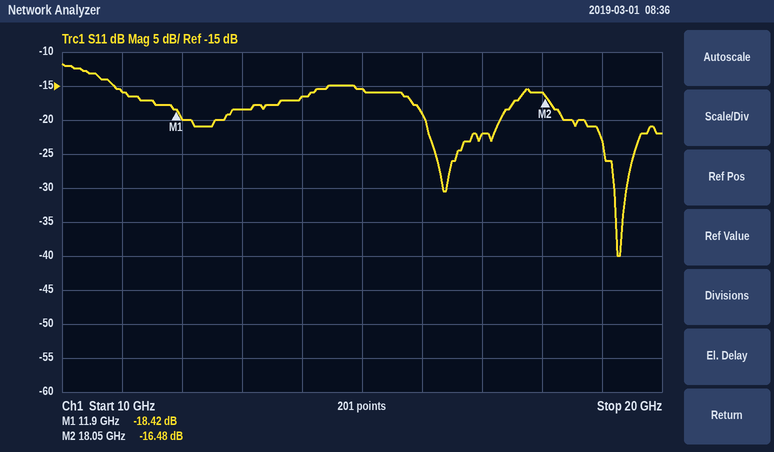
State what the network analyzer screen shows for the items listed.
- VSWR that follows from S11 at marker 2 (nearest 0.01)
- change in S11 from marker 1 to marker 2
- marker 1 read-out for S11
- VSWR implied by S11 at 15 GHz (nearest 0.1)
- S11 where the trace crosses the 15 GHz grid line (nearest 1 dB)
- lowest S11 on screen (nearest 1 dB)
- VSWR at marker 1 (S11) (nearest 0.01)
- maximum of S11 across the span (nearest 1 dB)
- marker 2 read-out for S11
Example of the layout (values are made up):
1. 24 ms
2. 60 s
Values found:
1. 1.35
2. 1.94 dB
3. -18.42 dB
4. 1.4
5. -15 dB
6. -40 dB
7. 1.27
8. -12 dB
9. -16.48 dB
